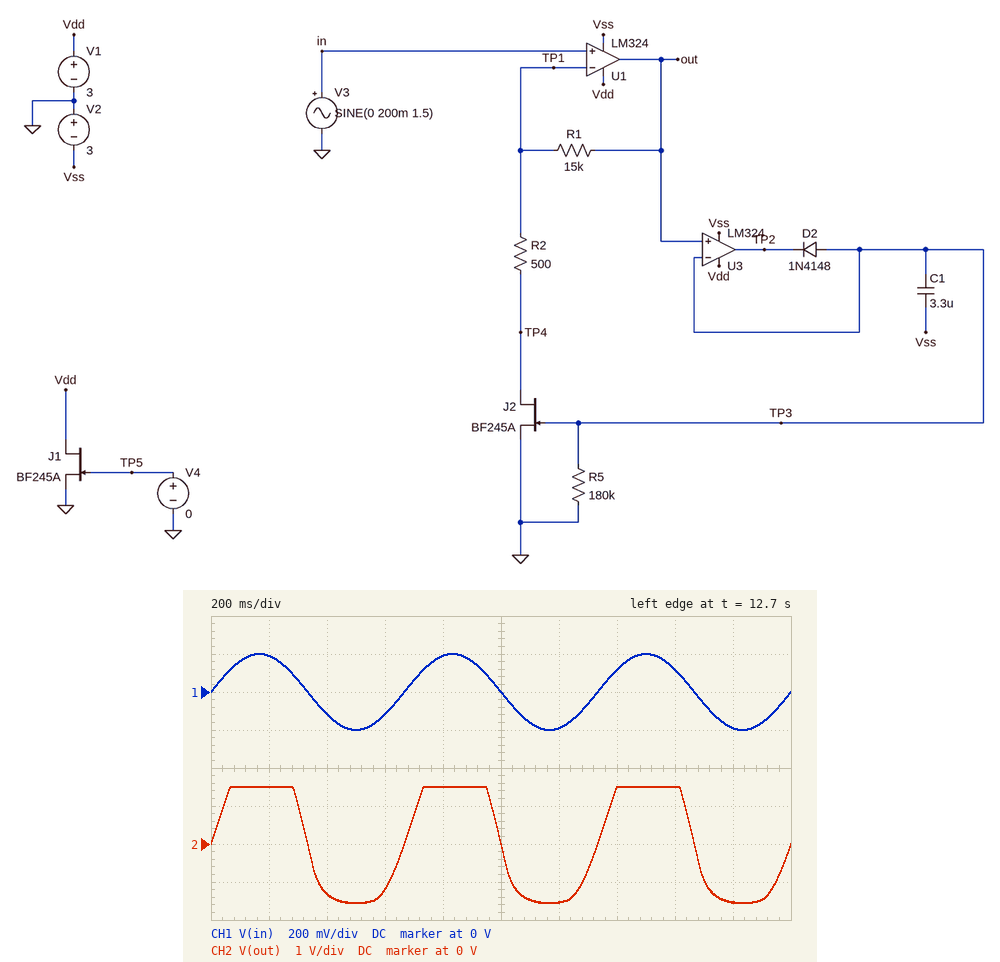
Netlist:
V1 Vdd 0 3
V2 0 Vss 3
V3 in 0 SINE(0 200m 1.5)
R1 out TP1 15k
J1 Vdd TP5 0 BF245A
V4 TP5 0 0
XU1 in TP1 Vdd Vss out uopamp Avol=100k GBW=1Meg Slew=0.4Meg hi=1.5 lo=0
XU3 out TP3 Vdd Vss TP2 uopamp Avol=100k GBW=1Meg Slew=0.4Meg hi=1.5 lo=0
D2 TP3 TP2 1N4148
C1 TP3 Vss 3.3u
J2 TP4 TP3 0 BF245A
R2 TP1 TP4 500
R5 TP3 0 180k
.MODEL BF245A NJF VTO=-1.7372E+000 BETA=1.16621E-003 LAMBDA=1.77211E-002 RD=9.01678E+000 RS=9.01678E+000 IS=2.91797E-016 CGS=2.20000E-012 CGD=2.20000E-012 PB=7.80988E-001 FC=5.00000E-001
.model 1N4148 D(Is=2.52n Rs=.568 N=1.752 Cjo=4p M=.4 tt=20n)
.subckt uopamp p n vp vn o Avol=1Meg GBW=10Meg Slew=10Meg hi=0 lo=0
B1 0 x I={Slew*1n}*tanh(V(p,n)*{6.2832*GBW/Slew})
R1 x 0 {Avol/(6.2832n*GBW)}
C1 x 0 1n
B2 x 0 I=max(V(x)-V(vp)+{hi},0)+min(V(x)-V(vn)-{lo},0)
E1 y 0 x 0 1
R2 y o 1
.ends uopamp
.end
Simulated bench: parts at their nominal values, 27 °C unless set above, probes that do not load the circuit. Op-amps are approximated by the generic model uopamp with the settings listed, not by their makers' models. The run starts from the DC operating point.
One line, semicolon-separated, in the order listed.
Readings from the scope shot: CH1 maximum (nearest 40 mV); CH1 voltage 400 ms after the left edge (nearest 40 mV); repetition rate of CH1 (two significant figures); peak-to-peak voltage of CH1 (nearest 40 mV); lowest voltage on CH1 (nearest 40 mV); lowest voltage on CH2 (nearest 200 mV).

200 mV; -120 mV; 1.5 Hz; 400 mV; -200 mV; -1.6 V
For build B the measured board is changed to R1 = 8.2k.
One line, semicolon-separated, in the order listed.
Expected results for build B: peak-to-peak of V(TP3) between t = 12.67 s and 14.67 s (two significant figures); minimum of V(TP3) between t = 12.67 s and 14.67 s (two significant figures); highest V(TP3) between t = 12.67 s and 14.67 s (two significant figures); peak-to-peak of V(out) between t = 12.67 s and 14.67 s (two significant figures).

770 mV; -1.3 V; -570 mV; 2.8 V
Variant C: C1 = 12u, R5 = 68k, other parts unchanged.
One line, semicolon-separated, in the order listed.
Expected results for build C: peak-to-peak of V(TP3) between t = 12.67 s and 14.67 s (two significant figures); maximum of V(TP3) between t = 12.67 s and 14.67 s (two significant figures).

720 mV; -840 mV
